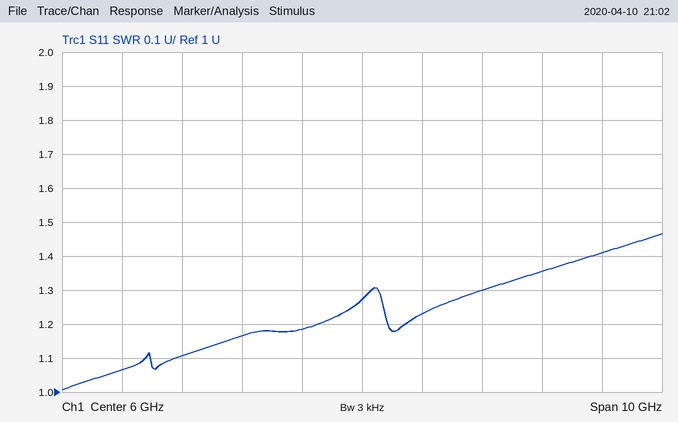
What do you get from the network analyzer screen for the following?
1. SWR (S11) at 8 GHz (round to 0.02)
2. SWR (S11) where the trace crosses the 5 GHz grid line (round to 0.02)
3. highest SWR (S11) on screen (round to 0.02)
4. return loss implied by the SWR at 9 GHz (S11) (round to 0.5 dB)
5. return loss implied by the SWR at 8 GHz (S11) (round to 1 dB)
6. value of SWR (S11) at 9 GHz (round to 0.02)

1.30
1.18
1.46
16.5 dB
18 dB
1.36
